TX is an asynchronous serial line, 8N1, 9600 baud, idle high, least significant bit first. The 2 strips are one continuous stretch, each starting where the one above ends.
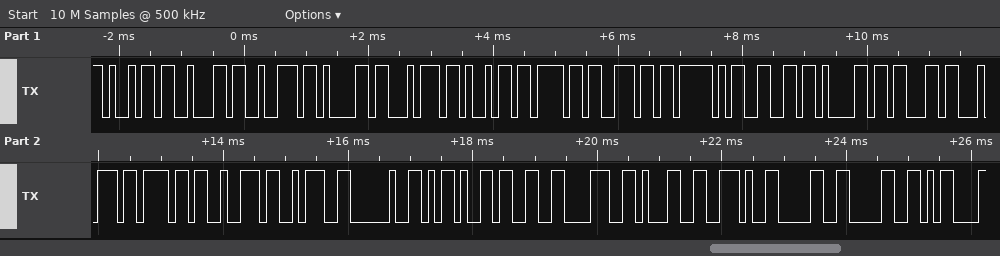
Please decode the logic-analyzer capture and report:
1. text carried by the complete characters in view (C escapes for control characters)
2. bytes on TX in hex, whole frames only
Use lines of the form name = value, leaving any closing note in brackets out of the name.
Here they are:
text carried by the complete characters in view = "ibration_factor: -381.00\r"
bytes on TX in hex, whole frames only = 69 62 72 61 74 69 6F 6E 5F 66 61 63 74 6F 72 3A 20 2D 33 38 31 2E 30 30 0D
